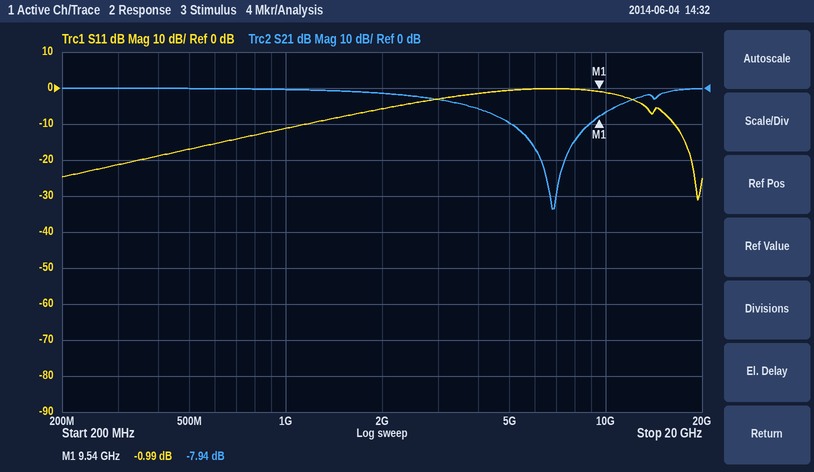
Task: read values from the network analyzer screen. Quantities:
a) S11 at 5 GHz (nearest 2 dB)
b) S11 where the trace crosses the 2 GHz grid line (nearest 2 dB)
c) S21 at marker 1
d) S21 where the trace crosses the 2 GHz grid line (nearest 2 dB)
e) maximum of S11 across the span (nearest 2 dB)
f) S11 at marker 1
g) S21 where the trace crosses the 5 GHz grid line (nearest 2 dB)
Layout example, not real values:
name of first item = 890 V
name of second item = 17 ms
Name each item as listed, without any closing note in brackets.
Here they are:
S11 at 5 GHz = 0 dB
S11 where the trace crosses the 2 GHz grid line = -6 dB
S21 at marker 1 = -7.94 dB
S21 where the trace crosses the 2 GHz grid line = -2 dB
maximum of S11 across the span = 0 dB
S11 at marker 1 = -0.99 dB
S21 where the trace crosses the 5 GHz grid line = -10 dB
